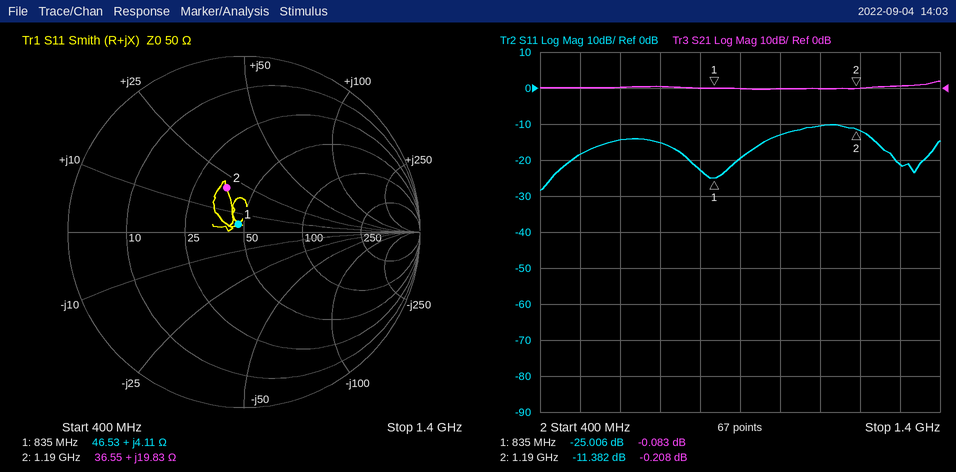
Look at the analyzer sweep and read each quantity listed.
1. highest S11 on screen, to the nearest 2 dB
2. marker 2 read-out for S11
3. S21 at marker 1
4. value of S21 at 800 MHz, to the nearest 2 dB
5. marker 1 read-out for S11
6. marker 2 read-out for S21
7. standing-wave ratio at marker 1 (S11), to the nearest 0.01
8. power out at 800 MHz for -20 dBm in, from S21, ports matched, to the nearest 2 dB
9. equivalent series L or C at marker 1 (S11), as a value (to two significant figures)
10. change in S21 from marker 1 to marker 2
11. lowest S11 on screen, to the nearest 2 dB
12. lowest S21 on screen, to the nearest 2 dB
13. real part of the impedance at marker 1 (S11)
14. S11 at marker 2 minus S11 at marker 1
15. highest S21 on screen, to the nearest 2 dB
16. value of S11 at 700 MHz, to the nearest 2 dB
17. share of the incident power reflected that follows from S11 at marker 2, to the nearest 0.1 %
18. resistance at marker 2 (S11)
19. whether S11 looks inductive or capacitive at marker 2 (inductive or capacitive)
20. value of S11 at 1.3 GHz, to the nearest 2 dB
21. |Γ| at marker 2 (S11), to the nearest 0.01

-10 dB
-11.382 dB
-0.083 dB
0 dB
-25.006 dB
-0.208 dB
1.12
-20 dBm
780 pH
-0.125 dB
-28 dB
0 dB
46.53 Ω
13.624 dB
2 dB
-16 dB
7.3 %
36.55 Ω
inductive
-22 dB
0.27
